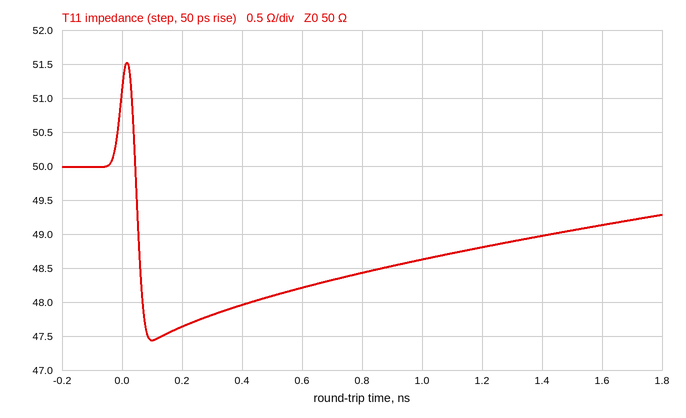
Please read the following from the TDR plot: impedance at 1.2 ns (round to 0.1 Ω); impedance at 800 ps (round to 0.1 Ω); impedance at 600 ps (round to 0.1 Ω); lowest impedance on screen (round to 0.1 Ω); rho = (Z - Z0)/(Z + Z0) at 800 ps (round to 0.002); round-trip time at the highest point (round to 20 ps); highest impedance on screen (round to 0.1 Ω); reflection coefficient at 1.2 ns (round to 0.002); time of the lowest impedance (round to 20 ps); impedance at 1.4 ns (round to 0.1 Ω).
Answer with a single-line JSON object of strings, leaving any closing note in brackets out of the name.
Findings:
{"impedance at 1.2 ns": "48.8 Ω", "impedance at 800 ps": "48.4 Ω", "impedance at 600 ps": "48.2 Ω", "lowest impedance on screen": "47.4 Ω", "rho = (Z - Z0)/(Z + Z0) at 800 ps": "-0.016", "round-trip time at the highest point": "20 ps", "highest impedance on screen": "51.5 Ω", "reflection coefficient at 1.2 ns": "-0.012", "time of the lowest impedance": "100 ps", "impedance at 1.4 ns": "49.0 Ω"}
